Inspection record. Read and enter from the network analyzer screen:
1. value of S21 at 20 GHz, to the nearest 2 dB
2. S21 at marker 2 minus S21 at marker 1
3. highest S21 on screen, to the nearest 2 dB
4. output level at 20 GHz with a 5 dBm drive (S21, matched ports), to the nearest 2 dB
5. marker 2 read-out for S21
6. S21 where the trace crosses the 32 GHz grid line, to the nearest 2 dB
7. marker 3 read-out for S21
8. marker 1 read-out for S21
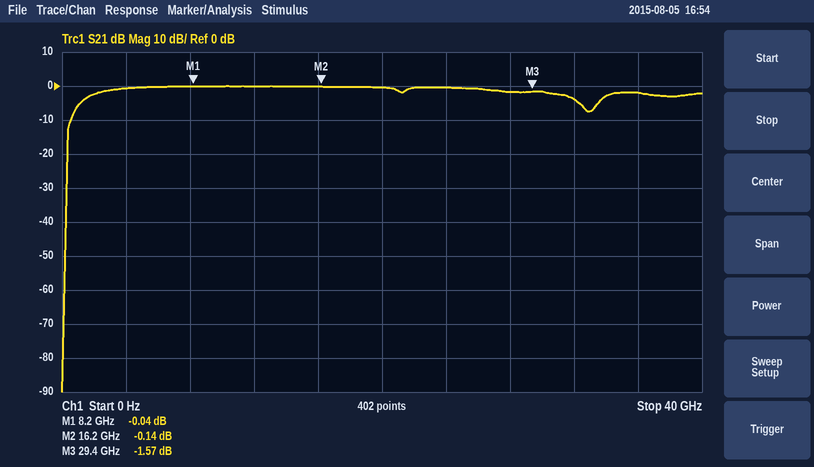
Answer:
0 dB
-0.10 dB
0 dB
4 dBm
-0.14 dB
-4 dB
-1.57 dB
-0.04 dB
